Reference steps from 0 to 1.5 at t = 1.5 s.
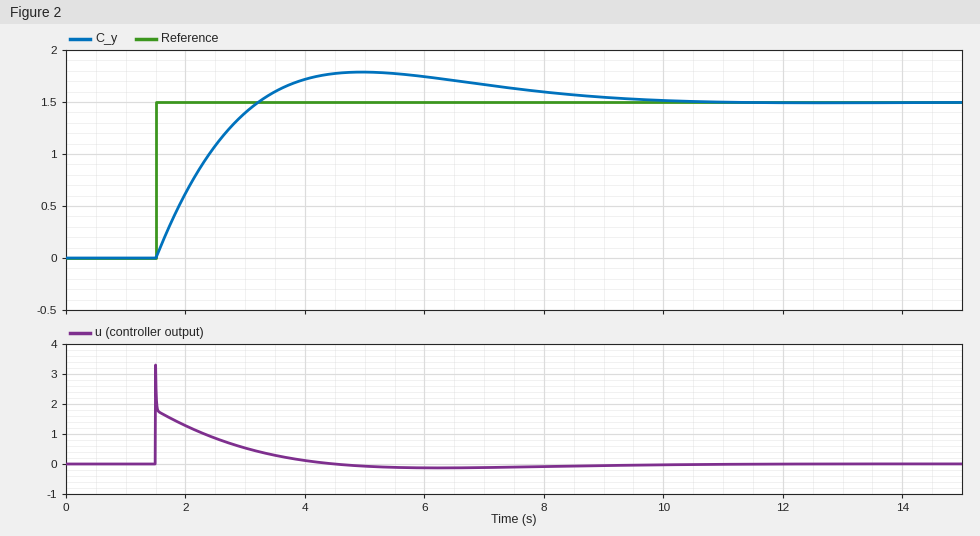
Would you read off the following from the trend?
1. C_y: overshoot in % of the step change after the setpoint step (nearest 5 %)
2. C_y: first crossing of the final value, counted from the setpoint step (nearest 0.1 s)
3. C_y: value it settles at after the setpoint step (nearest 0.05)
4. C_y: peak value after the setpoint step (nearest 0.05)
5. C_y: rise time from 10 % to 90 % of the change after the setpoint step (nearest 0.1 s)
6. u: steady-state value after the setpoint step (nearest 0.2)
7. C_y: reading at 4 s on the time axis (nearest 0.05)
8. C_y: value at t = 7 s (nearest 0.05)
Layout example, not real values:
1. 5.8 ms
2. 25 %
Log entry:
1. 20 %
2. 1.7 s
3. 1.50
4. 1.80
5. 1.3 s
6. 0.0
7. 1.70
8. 1.65
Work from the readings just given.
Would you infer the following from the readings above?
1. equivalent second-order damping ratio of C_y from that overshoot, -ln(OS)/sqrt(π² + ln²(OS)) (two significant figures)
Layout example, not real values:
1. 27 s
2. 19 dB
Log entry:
1. 0.46
